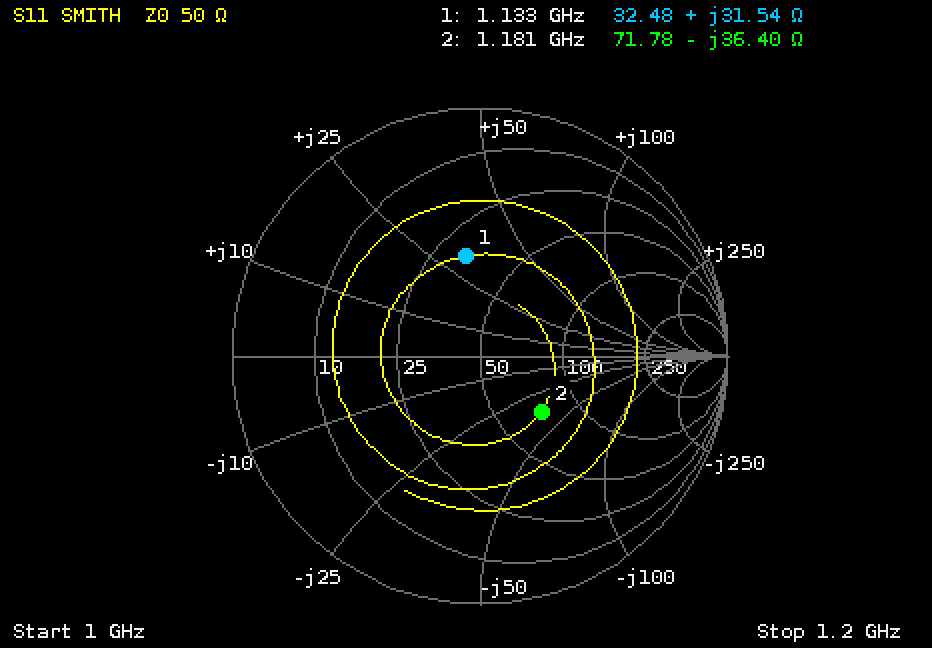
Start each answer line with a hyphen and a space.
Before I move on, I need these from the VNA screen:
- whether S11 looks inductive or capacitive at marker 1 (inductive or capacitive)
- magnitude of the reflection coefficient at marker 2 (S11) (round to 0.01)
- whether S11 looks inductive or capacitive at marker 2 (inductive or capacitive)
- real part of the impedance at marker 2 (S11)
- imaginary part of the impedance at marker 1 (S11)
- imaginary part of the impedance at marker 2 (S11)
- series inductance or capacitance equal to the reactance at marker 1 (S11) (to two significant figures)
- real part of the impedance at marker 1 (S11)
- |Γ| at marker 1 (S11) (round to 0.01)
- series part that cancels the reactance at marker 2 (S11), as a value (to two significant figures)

- inductive
- 0.33
- capacitive
- 71.78 Ω
- +31.54 Ω
- -36.40 Ω
- 4.4 nH
- 32.48 Ω
- 0.41
- 4.9 nH
